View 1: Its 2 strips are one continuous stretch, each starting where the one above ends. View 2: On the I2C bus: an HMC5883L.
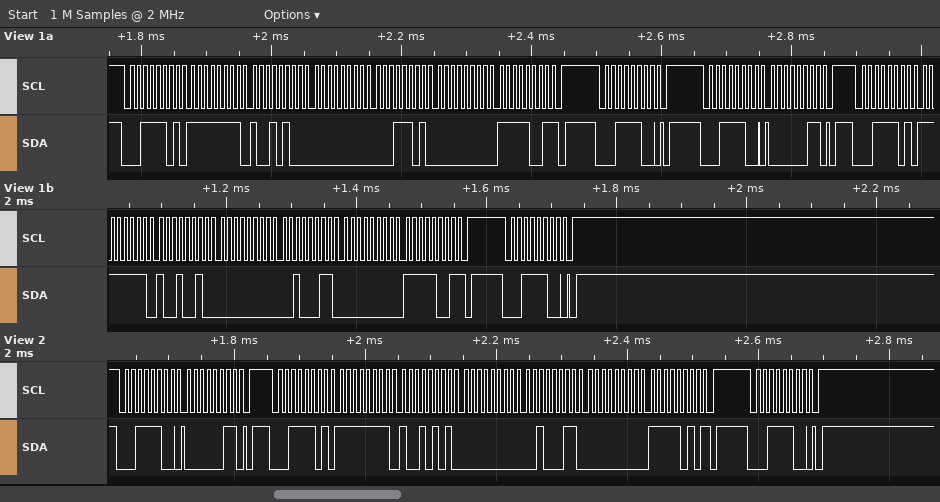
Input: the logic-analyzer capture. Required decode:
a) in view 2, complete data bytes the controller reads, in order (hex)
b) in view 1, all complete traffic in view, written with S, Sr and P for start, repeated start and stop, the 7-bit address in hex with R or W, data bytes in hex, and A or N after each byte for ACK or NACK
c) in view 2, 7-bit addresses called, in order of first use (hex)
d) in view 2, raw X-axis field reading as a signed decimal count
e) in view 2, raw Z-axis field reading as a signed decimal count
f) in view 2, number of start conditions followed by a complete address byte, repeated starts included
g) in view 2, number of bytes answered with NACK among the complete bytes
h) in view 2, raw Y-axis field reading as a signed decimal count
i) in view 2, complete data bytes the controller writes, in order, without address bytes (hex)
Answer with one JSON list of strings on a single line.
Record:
["FF 95 00 23 00 FA", "S 1ER A FF A 94 A 00 A 1D A 00 A F9 N P S 1EW A P S 1EW A 03 A P S 1ER A FF A 92 A 00 A 23 A 00 A F9 N P S 1EW A P", "0x1E", "-107", "35", "3", "1", "250", "03"]
